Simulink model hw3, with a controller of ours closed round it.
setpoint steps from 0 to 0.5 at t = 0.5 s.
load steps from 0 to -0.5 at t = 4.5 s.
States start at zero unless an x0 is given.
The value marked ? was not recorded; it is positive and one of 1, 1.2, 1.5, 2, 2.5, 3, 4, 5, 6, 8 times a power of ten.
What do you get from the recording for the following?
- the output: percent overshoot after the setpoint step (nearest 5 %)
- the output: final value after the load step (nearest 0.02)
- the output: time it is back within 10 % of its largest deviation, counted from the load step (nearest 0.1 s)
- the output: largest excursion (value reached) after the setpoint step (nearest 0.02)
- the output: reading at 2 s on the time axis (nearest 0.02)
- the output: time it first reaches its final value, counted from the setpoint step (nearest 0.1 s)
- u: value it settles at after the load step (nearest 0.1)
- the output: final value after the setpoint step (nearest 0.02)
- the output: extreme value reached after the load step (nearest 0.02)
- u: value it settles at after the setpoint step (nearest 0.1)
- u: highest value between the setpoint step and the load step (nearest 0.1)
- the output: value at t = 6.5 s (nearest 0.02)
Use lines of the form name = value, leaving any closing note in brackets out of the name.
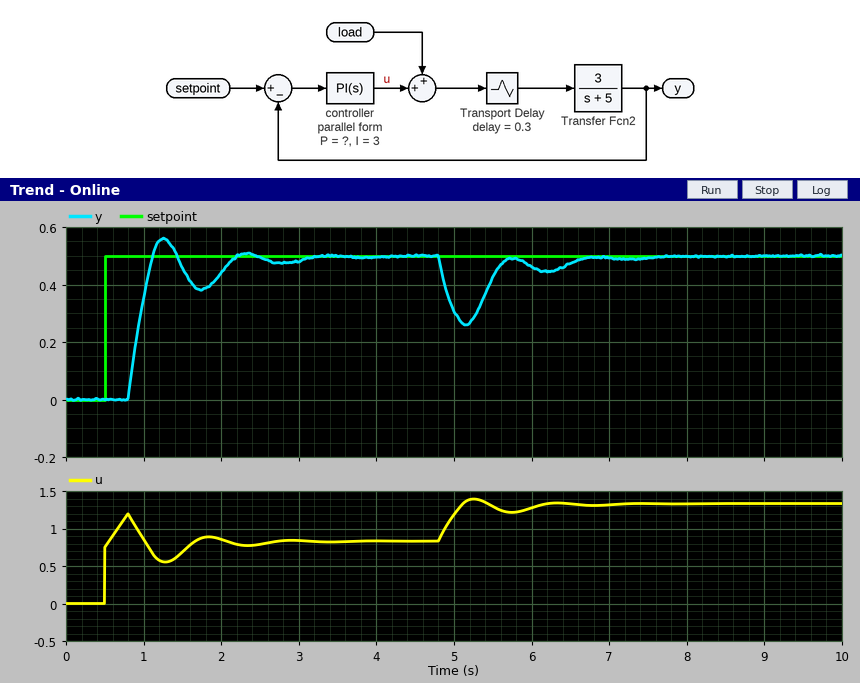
the output: percent overshoot after the setpoint step = 10 %
the output: final value after the load step = 0.50
the output: time it is back within 10 % of its largest deviation, counted from the load step = 2.0 s
the output: largest excursion (value reached) after the setpoint step = 0.56
the output: reading at 2 s on the time axis = 0.44
the output: time it first reaches its final value, counted from the setpoint step = 0.6 s
u: value it settles at after the load step = 1.3
the output: final value after the setpoint step = 0.50
the output: extreme value reached after the load step = 0.26
u: value it settles at after the setpoint step = 0.8
u: highest value between the setpoint step and the load step = 1.2
the output: value at t = 6.5 s = 0.48
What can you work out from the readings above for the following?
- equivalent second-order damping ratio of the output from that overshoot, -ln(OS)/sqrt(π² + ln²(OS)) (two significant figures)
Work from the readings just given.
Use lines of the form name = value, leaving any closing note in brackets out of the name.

equivalent second-order damping ratio of the output from that overshoot, -ln(OS)/sqrt(π² + ln²(OS)) = 0.59
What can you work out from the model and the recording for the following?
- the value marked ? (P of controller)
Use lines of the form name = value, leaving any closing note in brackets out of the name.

the value marked ? = 1.5
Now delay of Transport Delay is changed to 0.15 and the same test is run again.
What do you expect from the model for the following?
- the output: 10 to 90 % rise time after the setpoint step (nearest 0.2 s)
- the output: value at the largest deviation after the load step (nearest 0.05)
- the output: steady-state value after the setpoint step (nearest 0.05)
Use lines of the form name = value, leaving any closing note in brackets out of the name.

the output: 10 to 90 % rise time after the setpoint step = 1.2 s
the output: value at the largest deviation after the load step = 0.30
the output: steady-state value after the setpoint step = 0.50
